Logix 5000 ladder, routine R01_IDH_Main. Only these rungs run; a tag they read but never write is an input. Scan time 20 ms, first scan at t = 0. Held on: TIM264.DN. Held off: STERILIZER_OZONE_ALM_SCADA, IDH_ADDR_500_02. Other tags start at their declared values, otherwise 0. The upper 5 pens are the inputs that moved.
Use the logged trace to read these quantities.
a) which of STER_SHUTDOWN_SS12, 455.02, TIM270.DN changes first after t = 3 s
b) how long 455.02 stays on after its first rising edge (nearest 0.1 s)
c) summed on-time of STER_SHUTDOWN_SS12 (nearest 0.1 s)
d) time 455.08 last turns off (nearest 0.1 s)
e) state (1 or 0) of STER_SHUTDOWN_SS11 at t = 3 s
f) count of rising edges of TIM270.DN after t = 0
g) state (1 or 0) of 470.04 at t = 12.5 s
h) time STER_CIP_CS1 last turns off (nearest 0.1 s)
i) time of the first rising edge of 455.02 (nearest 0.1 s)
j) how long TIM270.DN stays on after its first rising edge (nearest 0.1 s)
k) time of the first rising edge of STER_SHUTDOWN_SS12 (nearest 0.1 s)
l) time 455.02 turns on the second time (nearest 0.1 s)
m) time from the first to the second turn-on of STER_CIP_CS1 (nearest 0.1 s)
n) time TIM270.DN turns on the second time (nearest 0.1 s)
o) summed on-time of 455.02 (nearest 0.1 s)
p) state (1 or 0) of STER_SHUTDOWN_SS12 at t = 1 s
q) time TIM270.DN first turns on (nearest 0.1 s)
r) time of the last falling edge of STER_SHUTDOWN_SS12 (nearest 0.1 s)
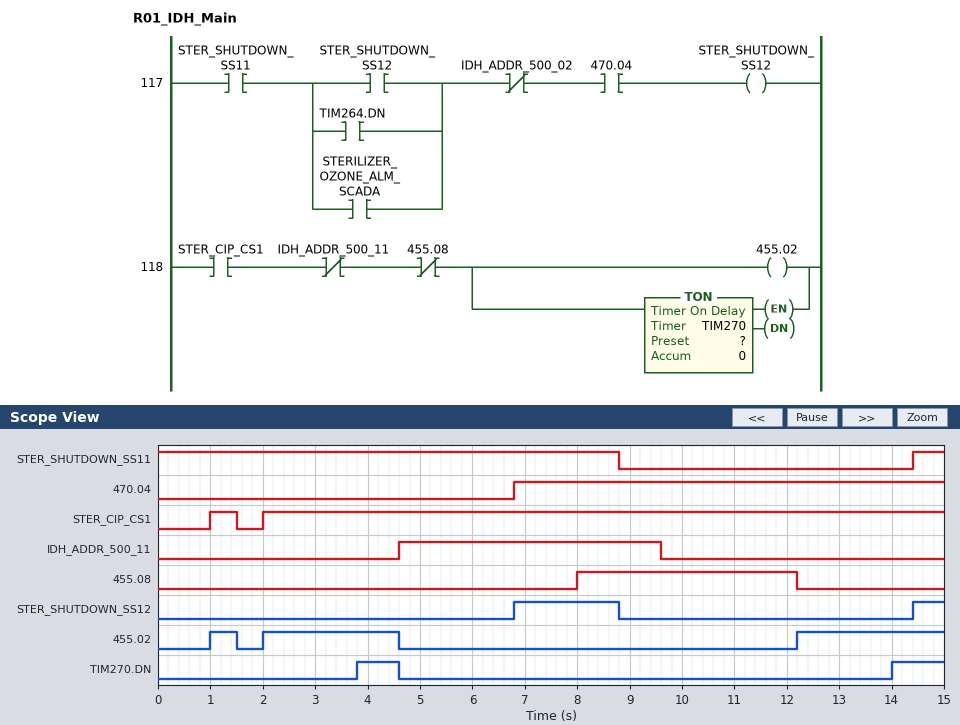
TIM270.DN
0.5 s
2.6 s
12.2 s
1
2
1
1.5 s
1.0 s
0.8 s
6.8 s
2.0 s
1.0 s
14.0 s
5.9 s
0
3.8 s
8.8 s
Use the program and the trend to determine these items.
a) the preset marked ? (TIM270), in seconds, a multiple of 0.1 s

1.8 s
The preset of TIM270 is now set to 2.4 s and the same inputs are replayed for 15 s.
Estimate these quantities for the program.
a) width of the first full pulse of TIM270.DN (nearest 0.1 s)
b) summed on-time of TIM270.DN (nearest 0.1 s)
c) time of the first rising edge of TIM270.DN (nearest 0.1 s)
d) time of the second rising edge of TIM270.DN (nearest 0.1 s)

0.2 s
0.6 s
4.4 s
14.6 s
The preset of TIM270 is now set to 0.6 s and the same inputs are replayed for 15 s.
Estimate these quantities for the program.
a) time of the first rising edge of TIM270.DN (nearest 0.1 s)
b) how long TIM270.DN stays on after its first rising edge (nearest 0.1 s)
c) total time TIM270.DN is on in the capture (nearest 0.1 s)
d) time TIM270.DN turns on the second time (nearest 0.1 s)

2.6 s
2.0 s
4.2 s
12.8 s
